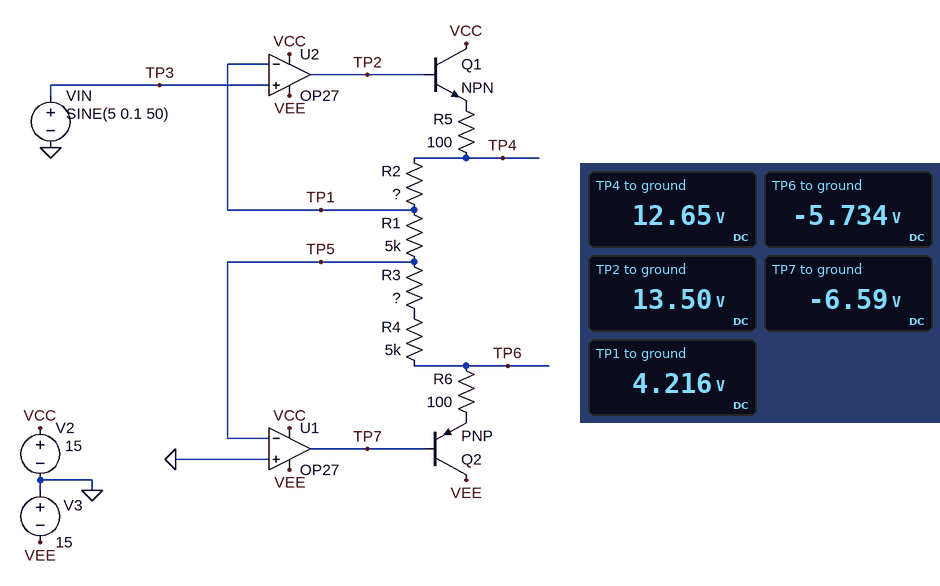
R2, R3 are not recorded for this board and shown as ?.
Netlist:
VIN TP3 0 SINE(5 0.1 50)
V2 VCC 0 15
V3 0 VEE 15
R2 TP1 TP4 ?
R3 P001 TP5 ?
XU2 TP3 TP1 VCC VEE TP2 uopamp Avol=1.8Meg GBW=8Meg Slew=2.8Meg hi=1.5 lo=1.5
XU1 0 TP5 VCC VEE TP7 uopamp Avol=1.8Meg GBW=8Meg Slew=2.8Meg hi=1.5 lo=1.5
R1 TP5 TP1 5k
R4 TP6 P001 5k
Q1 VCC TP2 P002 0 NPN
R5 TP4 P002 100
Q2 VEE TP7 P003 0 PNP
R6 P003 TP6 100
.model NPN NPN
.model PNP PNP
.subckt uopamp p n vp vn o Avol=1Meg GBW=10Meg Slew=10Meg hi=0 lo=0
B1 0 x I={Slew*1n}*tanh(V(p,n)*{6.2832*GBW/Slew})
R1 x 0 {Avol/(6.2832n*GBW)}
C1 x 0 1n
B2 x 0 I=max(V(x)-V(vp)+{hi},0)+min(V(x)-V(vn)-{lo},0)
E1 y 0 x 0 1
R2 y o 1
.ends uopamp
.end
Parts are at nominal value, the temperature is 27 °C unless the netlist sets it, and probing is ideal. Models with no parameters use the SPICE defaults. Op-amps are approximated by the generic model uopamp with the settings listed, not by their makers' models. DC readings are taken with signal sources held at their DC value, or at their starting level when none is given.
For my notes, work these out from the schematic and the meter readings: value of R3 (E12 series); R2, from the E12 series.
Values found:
1.8 kΩ
10 kΩ
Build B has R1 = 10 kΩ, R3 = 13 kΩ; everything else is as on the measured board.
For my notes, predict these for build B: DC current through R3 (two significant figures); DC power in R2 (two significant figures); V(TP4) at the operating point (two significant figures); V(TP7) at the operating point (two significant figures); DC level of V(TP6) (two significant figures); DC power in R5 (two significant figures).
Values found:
500 µA
2.5 mW
10 V
-9.8 V
-9.0 V
25 µW
